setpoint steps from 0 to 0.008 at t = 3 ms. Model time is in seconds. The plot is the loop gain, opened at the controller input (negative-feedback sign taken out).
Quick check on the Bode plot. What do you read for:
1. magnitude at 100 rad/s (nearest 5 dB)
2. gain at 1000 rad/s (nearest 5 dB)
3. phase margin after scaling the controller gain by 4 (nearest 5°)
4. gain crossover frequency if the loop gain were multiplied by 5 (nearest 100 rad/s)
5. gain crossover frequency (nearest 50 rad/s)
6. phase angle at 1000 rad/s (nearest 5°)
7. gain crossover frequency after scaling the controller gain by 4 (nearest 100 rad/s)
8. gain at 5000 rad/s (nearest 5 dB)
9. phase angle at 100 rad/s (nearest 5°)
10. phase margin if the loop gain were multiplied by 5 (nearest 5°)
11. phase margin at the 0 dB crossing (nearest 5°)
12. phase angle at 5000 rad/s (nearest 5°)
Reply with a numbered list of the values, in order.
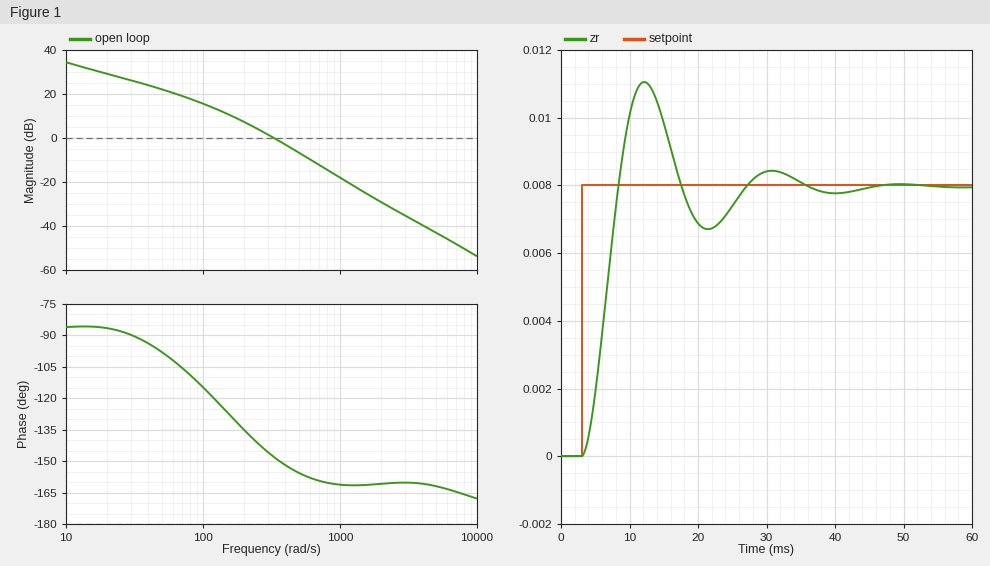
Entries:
1. 15 dB
2. -20 dB
3. 20°
4. 800 rad/s
5. 350 rad/s
6. -160°
7. 700 rad/s
8. -45 dB
9. -115°
10. 20°
11. 30°
12. -160°
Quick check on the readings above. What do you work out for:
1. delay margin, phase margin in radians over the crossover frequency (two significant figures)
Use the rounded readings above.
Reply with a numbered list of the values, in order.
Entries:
1. 0.0015 s
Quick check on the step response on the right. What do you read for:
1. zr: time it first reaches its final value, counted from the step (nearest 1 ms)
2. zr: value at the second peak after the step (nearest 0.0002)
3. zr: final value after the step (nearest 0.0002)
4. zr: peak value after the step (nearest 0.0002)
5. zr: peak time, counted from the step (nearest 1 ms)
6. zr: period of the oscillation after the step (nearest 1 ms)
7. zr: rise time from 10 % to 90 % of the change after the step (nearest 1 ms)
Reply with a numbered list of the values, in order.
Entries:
1. 5 ms
2. 0.0084
3. 0.0080
4. 0.0110
5. 9 ms
6. 19 ms
7. 4 ms
